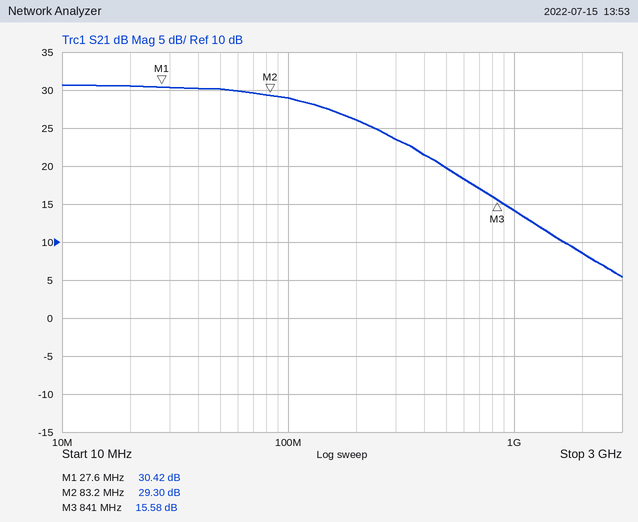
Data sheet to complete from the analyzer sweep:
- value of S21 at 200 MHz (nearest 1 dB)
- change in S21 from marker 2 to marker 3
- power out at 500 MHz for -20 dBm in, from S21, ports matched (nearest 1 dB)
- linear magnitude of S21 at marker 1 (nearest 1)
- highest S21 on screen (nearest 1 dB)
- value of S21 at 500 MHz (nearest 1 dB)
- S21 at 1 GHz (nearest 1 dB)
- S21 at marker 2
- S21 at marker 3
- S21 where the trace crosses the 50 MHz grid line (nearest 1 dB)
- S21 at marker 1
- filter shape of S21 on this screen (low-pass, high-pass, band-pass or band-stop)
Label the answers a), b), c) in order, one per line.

a) 26 dB
b) -13.72 dB
c) 0 dBm
d) 33
e) 31 dB
f) 20 dB
g) 14 dB
h) 29.30 dB
i) 15.58 dB
j) 30 dB
k) 30.42 dB
l) low-pass
